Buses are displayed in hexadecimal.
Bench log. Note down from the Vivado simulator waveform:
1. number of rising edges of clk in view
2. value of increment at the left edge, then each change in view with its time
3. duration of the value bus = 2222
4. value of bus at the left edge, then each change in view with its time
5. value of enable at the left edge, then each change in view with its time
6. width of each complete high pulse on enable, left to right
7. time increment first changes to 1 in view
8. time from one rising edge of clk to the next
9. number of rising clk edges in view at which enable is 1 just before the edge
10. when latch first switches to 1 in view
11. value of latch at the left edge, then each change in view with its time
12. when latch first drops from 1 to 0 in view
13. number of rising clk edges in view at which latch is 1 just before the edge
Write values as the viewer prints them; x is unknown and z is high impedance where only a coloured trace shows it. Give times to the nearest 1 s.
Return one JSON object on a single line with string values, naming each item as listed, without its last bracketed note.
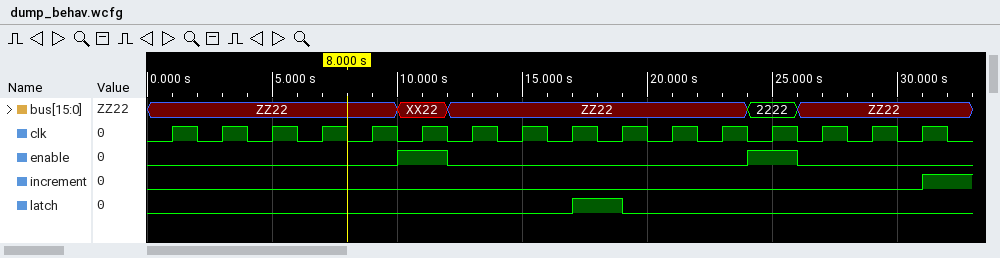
{"number of rising edges of clk in view": "16", "value of increment at the left edge, then each change in view with its time": "0, 1 at 31 s", "duration of the value bus = 2222": "2 s", "value of bus at the left edge, then each change in view with its time": "ZZ22, XX22 at 10 s, ZZ22 at 12 s, 2222 at 24 s, ZZ22 at 26 s", "value of enable at the left edge, then each change in view with its time": "0, 1 at 10 s, 0 at 12 s, 1 at 24 s, 0 at 26 s", "width of each complete high pulse on enable, left to right": "2 s, 2 s", "time increment first changes to 1 in view": "31 s", "time from one rising edge of clk to the next": "2 s", "number of rising clk edges in view at which enable is 1 just before the edge": "2", "when latch first switches to 1 in view": "17 s", "value of latch at the left edge, then each change in view with its time": "0, 1 at 17 s, 0 at 19 s", "when latch first drops from 1 to 0 in view": "19 s", "number of rising clk edges in view at which latch is 1 just before the edge": "1"}
